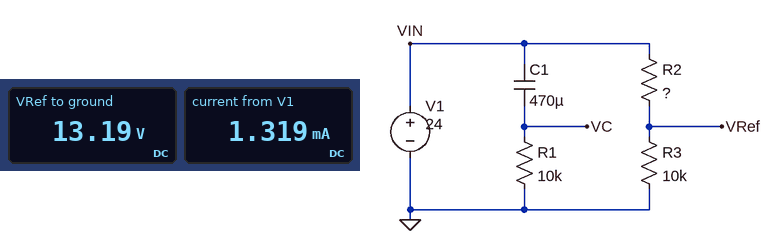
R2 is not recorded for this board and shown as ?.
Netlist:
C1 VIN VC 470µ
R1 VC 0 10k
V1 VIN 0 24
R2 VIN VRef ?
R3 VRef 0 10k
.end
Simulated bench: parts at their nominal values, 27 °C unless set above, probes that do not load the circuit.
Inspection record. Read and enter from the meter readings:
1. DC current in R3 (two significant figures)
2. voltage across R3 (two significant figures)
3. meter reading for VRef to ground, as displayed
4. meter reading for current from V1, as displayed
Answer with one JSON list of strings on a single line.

["1.3 mA", "13 V", "13.19 V", "1.319 mA"]
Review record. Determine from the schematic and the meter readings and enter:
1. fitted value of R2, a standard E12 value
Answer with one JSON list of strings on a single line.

["8.2 kΩ"]
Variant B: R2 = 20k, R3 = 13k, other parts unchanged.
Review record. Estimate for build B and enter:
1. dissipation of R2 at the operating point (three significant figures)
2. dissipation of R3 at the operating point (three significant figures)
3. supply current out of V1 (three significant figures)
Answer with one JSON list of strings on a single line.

["10.6 mW", "6.88 mW", "727 µA"]
